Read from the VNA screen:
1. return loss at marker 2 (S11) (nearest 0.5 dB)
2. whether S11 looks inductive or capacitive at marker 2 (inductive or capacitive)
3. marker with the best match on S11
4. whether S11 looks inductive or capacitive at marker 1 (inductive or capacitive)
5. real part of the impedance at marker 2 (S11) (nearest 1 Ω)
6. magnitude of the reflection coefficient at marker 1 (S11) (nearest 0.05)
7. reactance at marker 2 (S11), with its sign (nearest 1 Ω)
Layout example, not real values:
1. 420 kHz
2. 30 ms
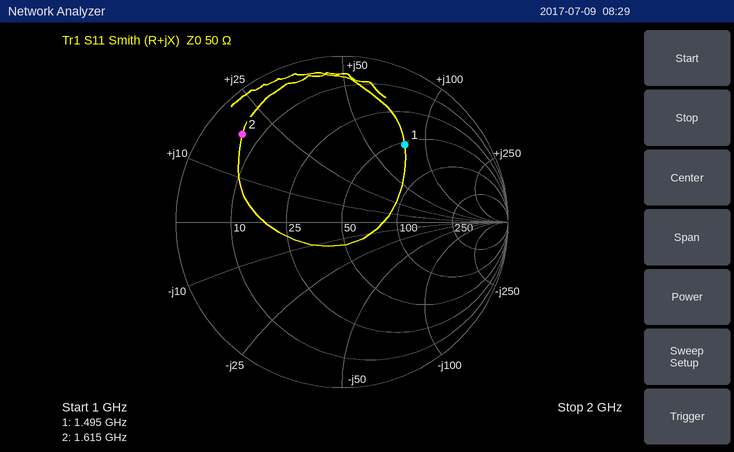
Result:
1. 2.0 dB
2. inductive
3. marker 1
4. inductive
5. 6 Ω
6. 0.60
7. +19 Ω
